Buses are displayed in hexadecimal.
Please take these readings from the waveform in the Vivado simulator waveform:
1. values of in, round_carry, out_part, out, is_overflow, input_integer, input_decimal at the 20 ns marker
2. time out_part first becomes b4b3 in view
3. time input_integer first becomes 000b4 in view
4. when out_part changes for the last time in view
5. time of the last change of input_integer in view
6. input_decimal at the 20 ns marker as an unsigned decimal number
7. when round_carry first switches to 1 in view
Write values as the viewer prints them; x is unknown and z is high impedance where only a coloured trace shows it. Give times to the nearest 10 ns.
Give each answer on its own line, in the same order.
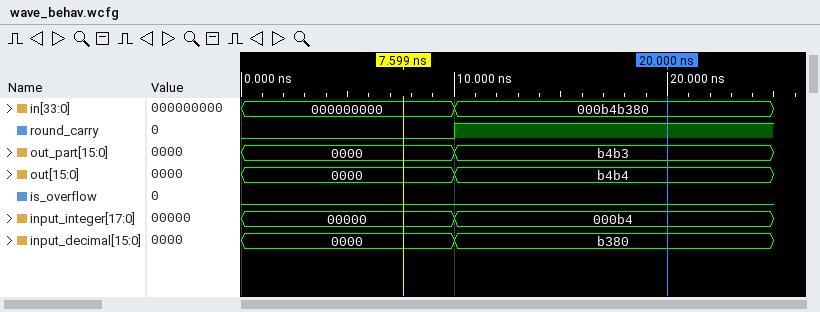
in=000b4b380, round_carry=1, out_part=b4b3, out=b4b4, is_overflow=0, input_integer=000b4, input_decimal=b380
10 ns
10 ns
10 ns
10 ns
45952
10 ns
